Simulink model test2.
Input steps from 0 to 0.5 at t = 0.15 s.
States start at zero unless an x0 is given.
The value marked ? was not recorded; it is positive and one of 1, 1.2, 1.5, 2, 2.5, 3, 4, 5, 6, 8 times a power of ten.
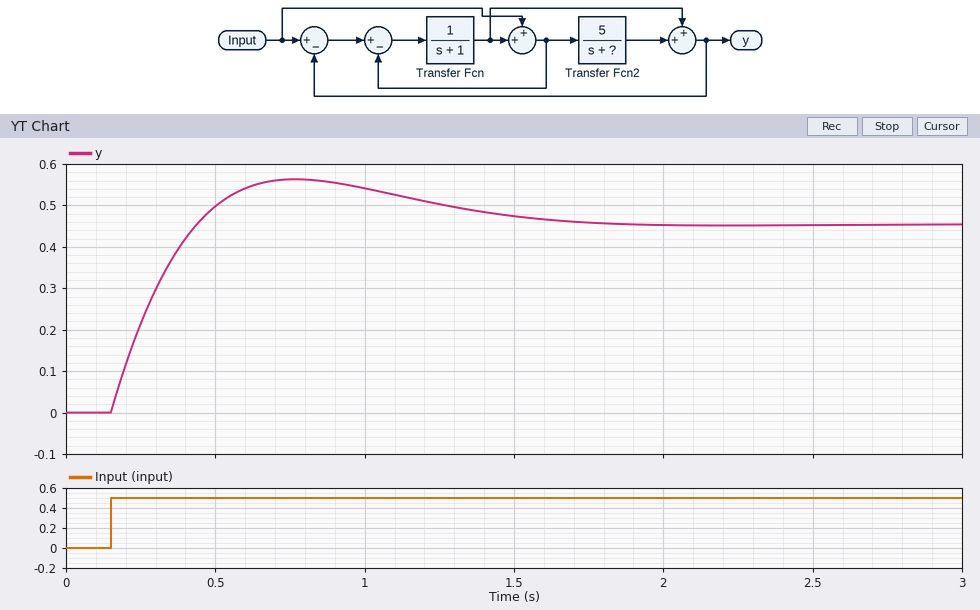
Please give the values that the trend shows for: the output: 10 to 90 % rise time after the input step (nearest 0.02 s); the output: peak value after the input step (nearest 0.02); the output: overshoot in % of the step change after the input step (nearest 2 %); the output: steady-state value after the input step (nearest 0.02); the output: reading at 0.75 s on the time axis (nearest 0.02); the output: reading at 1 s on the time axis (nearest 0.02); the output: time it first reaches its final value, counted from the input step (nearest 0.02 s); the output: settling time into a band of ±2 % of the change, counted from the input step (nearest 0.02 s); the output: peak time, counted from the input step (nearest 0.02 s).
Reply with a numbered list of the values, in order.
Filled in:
1. 0.22 s
2. 0.56
3. 24 %
4. 0.46
5. 0.56
6. 0.54
7. 0.28 s
8. 1.50 s
9. 0.62 s
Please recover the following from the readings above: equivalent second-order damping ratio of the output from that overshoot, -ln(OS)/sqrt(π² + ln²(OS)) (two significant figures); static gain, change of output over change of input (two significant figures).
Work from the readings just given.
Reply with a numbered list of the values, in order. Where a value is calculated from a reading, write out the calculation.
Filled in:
1. ln(0.24) = -1.427; 1.427 / sqrt(9.870 + 2.037) = 0.41
2. (0.46 - 0) / (0.5 - 0) = 0.92
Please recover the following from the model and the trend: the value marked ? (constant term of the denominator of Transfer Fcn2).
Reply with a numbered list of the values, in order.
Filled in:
1. 2
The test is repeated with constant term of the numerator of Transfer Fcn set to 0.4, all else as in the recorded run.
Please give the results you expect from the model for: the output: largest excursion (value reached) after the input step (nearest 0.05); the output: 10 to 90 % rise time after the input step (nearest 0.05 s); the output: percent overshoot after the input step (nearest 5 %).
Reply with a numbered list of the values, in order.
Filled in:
1. 0.75
2. 0.30 s
3. 20 %
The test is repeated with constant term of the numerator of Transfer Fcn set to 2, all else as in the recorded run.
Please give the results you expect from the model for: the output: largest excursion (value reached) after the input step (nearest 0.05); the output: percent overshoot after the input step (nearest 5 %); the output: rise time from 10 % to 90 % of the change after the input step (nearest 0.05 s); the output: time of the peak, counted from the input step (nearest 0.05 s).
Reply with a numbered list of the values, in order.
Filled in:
1. 0.45
2. 15 %
3. 0.20 s
4. 0.50 s
